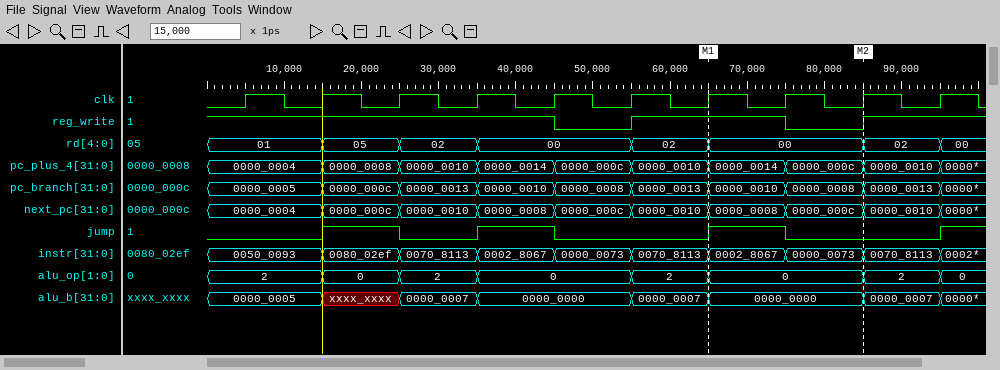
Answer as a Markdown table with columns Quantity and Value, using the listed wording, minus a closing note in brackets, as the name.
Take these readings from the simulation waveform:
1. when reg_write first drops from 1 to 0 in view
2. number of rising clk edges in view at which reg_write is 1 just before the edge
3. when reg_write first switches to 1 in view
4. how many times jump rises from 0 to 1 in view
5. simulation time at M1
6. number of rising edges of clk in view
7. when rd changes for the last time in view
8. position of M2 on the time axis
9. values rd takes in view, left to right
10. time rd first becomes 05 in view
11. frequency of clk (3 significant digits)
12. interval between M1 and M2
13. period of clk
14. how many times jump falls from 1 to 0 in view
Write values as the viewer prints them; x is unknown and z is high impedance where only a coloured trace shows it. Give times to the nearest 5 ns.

| Quantity | Value |
|---|---|
| when reg_write first drops from 1 to 0 in view | 45 ns |
| number of rising clk edges in view at which reg_write is 1 just before the edge | 8 |
| when reg_write first switches to 1 in view | 55 ns |
| how many times jump rises from 0 to 1 in view | 4 |
| simulation time at M1 | 65 ns |
| number of rising edges of clk in view | 10 |
| when rd changes for the last time in view | 95 ns |
| position of M2 on the time axis | 85 ns |
| values rd takes in view, left to right | 01, 05, 02, 00, 02, 00, 02, 00 |
| time rd first becomes 05 in view | 15 ns |
| frequency of clk | 100 MHz |
| interval between M1 and M2 | 20 ns |
| period of clk | 10 ns |
| how many times jump falls from 1 to 0 in view | 3 |
